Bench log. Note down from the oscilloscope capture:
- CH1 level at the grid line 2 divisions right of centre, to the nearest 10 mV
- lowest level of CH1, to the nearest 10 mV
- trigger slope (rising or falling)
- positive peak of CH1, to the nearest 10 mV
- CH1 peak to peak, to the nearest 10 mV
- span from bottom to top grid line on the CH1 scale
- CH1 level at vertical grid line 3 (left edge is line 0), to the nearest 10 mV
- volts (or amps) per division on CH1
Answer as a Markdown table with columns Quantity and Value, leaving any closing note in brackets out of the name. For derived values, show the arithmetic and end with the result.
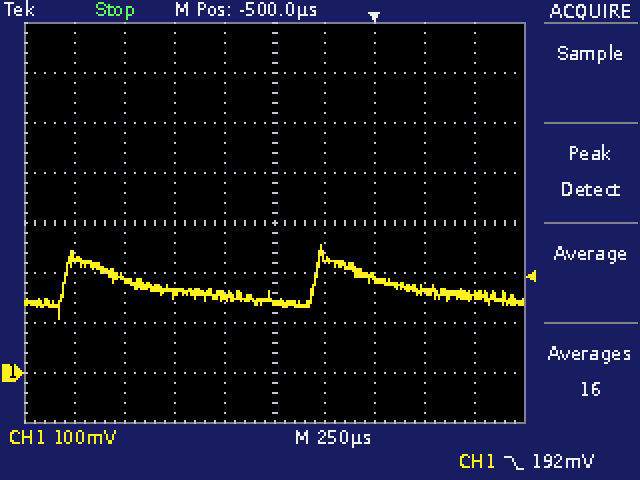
| Quantity | Value |
|---|---|
| CH1 level at the grid line 2 divisions right of centre, to the nearest 10 mV | 190 mV |
| lowest level of CH1, to the nearest 10 mV | 110 mV |
| trigger slope | falling |
| positive peak of CH1, to the nearest 10 mV | 260 mV |
| CH1 peak to peak, to the nearest 10 mV | 260 mV − (110 mV) = 150 mV |
| span from bottom to top grid line on the CH1 scale | 800 mV |
| CH1 level at vertical grid line 3 (left edge is line 0), to the nearest 10 mV | 160 mV |
| volts (or amps) per division on CH1 | 100 mV |
